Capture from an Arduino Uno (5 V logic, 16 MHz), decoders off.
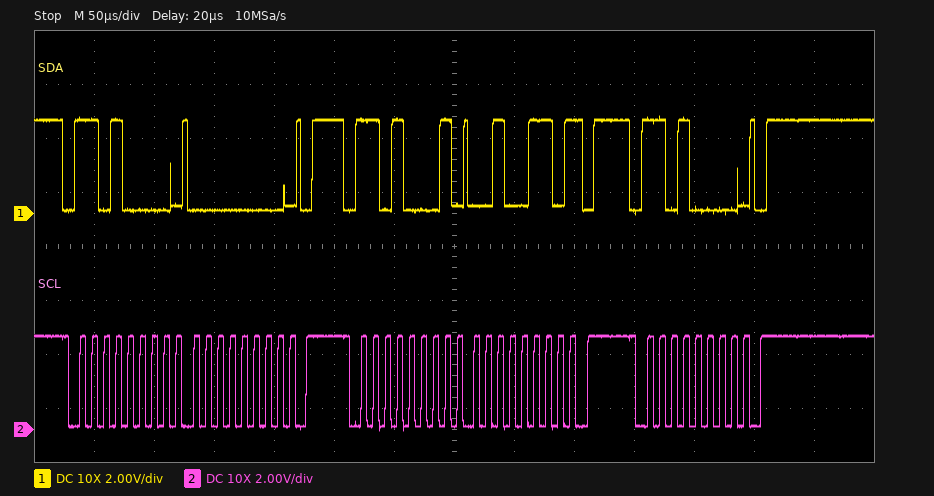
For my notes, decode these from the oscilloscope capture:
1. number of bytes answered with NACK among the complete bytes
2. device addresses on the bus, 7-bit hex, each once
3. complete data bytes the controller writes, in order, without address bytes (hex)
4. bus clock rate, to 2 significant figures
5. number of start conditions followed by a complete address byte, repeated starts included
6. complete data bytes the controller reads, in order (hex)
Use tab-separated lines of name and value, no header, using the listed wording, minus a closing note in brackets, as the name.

number of bytes answered with NACK among the complete bytes	1
device addresses on the bus, 7-bit hex, each once	0x68
complete data bytes the controller writes, in order, without address bytes	00
bus clock rate, to 2 significant figures	100 kHz
number of start conditions followed by a complete address byte, repeated starts included	3
complete data bytes the controller reads, in order	26
